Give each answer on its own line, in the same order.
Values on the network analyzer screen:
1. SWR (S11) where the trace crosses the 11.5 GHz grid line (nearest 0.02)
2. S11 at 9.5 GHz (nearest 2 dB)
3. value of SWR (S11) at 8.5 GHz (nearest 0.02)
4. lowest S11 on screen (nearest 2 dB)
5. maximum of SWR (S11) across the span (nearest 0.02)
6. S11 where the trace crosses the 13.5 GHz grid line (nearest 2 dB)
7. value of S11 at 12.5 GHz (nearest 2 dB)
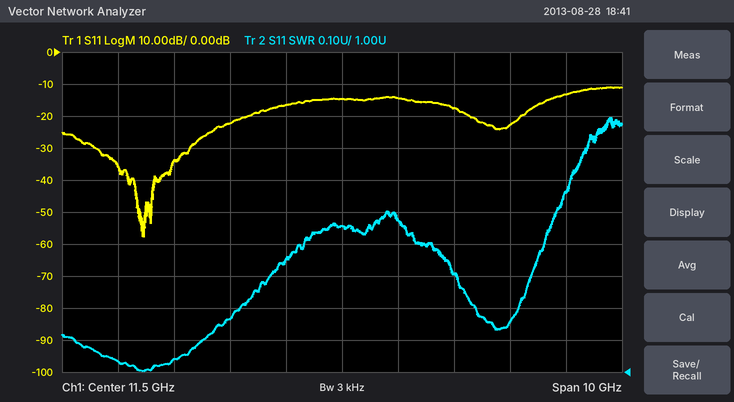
1.46
-22 dB
1.04
-58 dB
1.80
-18 dB
-14 dB
